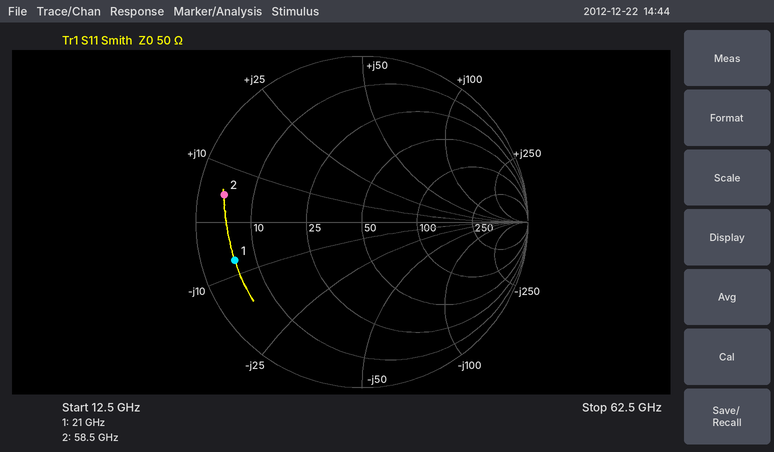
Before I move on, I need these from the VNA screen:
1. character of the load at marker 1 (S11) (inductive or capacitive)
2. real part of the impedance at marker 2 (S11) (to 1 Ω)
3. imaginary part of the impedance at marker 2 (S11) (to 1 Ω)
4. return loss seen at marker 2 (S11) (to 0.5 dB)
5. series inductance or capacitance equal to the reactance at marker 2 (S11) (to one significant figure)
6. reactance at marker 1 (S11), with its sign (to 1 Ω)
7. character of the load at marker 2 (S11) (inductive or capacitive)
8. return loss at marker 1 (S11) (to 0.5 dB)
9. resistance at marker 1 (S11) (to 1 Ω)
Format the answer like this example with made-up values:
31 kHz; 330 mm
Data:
capacitive; 4 Ω; +5 Ω; 1.5 dB; 10 pH; -7 Ω; inductive; 2.0 dB; 6 Ω
